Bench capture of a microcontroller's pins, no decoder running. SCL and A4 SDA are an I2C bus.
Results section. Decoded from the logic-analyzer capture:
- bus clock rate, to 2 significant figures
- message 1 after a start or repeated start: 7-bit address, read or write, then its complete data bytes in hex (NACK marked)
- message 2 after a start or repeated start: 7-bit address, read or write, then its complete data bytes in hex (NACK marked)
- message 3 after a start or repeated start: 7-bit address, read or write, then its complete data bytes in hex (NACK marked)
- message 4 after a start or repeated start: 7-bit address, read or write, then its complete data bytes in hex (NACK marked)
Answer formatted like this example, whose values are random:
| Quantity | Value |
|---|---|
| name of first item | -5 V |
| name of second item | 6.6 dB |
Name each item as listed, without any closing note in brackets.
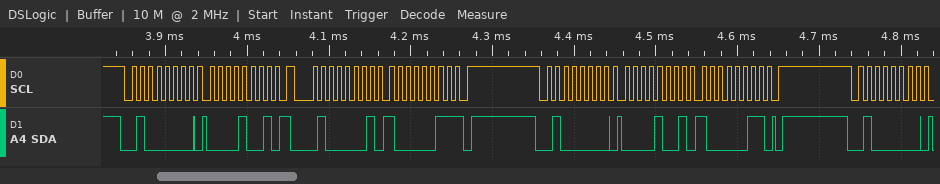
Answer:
| Quantity | Value |
|---|---|
| bus clock rate, to 2 significant figures | 100 kHz |
| message 1 after a start or repeated start: 7-bit address, read or write, then its complete data bytes in hex | 0x20 write: 09 |
| message 2 after a start or repeated start: 7-bit address, read or write, then its complete data bytes in hex | 0x20 read: 83 NACK |
| message 3 after a start or repeated start: 7-bit address, read or write, then its complete data bytes in hex | 0x20 write: 09 83 |
| message 4 after a start or repeated start: 7-bit address, read or write, then its complete data bytes in hex | 0x20 write |
